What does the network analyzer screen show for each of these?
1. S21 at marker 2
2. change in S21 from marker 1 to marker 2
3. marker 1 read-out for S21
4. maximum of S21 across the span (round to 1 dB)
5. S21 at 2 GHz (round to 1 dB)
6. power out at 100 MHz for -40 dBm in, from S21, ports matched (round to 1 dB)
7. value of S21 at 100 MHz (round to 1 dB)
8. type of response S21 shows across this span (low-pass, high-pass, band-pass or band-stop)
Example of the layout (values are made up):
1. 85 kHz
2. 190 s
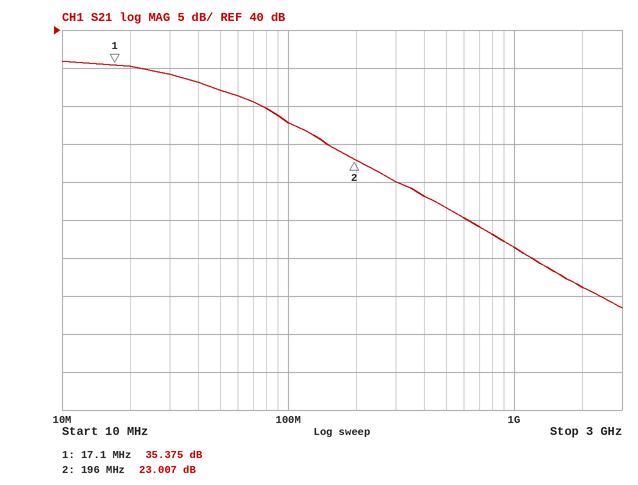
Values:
1. 23.007 dB
2. -12.368 dB
3. 35.375 dB
4. 36 dB
5. 6 dB
6. -12 dBm
7. 28 dB
8. low-pass
